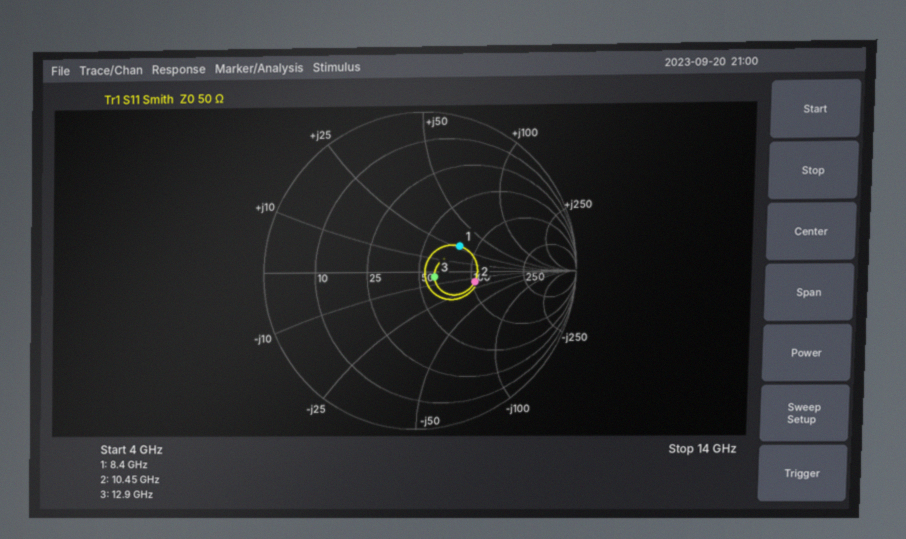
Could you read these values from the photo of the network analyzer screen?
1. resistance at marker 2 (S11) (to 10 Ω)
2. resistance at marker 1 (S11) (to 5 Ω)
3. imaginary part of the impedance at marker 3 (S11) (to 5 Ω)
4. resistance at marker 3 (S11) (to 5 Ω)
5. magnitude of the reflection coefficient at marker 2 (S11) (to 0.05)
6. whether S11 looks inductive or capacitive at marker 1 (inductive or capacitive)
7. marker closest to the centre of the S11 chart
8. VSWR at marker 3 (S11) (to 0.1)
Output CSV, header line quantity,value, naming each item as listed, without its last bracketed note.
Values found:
quantity,value
resistance at marker 2 (S11),100 Ω
resistance at marker 1 (S11),80 Ω
imaginary part of the impedance at marker 3 (S11),-5 Ω
resistance at marker 3 (S11),60 Ω
magnitude of the reflection coefficient at marker 2 (S11),0.35
whether S11 looks inductive or capacitive at marker 1,inductive
marker closest to the centre of the S11 chart,marker 3
VSWR at marker 3 (S11),1.2
